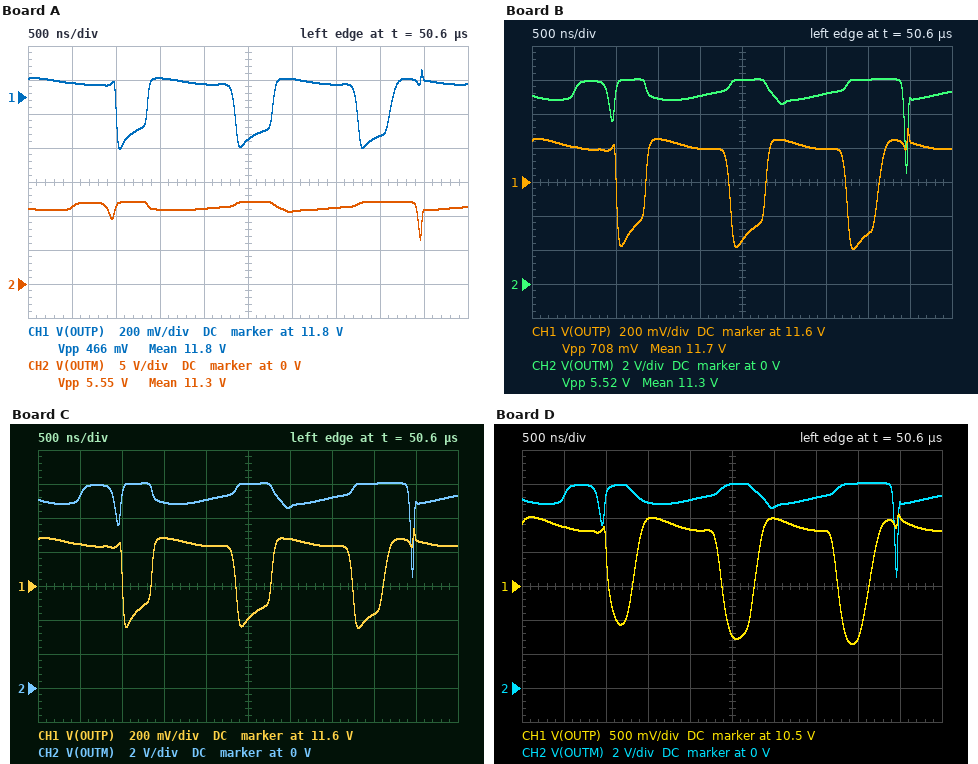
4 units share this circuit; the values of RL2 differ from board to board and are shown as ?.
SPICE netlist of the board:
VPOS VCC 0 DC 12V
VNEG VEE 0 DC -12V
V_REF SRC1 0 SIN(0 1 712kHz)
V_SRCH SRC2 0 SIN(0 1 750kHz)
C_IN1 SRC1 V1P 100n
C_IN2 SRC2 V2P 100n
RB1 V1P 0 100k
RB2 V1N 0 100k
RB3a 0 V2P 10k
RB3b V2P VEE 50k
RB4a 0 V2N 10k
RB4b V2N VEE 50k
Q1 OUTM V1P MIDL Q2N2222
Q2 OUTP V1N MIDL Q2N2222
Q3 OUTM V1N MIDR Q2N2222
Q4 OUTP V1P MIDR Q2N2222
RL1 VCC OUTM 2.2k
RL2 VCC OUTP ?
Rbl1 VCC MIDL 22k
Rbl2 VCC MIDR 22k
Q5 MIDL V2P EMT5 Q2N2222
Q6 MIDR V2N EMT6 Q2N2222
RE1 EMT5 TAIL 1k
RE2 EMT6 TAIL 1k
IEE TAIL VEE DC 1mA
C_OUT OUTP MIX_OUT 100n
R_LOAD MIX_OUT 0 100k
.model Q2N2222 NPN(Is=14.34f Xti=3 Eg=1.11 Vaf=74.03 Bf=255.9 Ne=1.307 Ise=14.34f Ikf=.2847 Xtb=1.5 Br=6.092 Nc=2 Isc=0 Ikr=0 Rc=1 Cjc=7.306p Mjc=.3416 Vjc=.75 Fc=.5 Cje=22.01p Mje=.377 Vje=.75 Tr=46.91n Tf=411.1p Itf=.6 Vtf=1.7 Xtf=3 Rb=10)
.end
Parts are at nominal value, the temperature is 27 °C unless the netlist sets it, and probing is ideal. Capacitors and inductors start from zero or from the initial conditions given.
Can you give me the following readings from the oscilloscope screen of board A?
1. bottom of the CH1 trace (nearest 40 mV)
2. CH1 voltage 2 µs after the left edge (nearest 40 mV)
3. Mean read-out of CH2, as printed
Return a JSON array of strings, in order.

["11.48 V", "11.88 V", "11.3 V"]
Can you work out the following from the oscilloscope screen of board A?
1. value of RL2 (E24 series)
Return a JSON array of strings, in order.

["910 Ω"]
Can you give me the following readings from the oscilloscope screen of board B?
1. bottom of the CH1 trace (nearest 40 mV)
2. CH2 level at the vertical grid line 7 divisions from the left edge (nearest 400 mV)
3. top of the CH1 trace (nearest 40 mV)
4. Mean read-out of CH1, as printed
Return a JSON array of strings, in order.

["11.20 V", "11.2 V", "11.92 V", "11.7 V"]
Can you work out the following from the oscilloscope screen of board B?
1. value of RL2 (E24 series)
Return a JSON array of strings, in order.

["1.5 kΩ"]
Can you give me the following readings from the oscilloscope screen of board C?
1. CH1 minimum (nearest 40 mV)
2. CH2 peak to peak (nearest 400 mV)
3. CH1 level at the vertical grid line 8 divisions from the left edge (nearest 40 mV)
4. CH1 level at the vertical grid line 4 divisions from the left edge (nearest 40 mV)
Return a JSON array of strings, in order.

["11.36 V", "5.6 V", "11.44 V", "11.84 V"]
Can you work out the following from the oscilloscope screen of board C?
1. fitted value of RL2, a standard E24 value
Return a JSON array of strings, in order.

["1.2 kΩ"]
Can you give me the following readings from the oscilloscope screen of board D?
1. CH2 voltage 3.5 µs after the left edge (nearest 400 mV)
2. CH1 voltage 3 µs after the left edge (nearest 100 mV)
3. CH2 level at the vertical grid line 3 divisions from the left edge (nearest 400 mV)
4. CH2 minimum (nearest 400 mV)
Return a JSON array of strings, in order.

["11.2 V", "11.5 V", "10.8 V", "6.4 V"]
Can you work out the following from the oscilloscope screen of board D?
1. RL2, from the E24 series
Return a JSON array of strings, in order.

["5.1 kΩ"]
